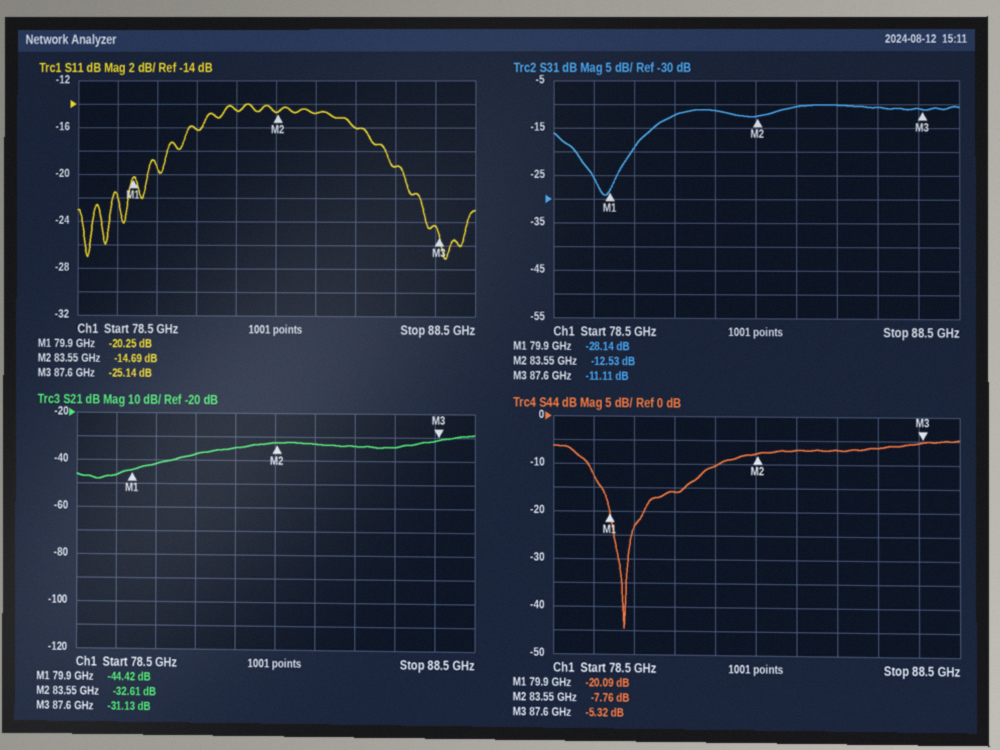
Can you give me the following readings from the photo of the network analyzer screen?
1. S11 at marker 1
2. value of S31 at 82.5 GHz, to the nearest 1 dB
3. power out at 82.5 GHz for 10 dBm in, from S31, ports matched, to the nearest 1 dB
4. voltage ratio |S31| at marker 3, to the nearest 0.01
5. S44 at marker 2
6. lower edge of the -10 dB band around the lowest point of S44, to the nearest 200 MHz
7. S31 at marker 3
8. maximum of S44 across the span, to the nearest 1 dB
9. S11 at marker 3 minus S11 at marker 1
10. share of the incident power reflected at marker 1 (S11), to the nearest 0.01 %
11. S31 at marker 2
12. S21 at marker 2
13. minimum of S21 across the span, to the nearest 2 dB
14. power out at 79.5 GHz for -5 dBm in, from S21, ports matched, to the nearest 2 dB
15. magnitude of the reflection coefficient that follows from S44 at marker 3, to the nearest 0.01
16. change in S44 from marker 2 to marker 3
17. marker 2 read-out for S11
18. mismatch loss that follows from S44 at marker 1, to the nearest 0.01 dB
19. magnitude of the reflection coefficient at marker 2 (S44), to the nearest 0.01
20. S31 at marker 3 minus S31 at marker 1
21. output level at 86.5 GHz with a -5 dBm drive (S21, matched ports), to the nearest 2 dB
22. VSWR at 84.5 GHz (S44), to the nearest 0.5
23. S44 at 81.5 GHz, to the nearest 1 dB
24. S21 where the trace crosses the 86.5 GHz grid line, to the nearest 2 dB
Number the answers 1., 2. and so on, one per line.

1. -20.25 dB
2. -11 dB
3. -1 dBm
4. 0.28
5. -7.76 dB
6. 79.4 GHz
7. -11.11 dB
8. -5 dB
9. -4.89 dB
10. 0.94 %
11. -12.53 dB
12. -32.61 dB
13. -48 dB
14. -52 dBm
15. 0.54
16. 2.44 dB
17. -14.69 dB
18. 0.04 dB
19. 0.41
20. 17.03 dB
21. -40 dBm
22. 2.5
23. -16 dB
24. -34 dB
